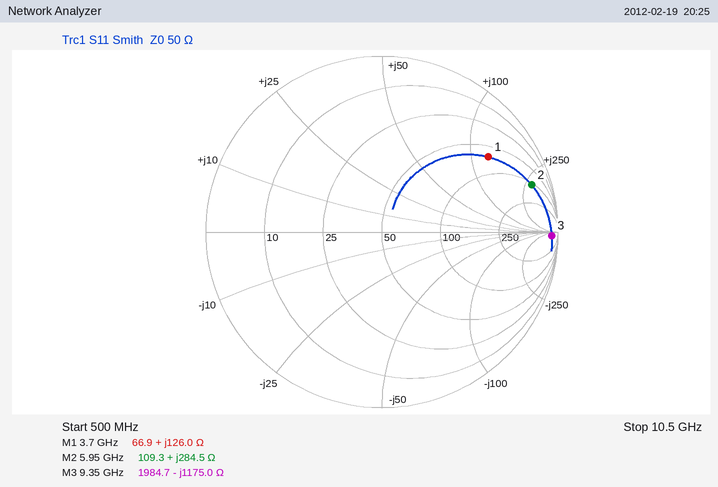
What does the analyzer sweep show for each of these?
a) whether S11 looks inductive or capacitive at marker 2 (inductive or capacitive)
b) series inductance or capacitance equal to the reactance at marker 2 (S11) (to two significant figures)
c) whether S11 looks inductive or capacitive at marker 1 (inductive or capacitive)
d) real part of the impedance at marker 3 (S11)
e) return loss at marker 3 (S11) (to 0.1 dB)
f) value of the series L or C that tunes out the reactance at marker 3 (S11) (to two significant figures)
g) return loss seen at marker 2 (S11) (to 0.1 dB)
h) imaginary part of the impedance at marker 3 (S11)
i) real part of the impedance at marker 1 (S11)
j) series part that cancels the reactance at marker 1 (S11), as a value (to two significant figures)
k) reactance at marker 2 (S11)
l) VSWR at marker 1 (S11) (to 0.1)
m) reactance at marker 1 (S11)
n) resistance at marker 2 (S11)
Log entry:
inductive
7.6 nH
inductive
1984.7 Ω
0.3 dB
20 nH
1.0 dB
-1175.0 Ω
66.9 Ω
340 fF
+284.5 Ω
6.7
+126.0 Ω
109.3 Ω
